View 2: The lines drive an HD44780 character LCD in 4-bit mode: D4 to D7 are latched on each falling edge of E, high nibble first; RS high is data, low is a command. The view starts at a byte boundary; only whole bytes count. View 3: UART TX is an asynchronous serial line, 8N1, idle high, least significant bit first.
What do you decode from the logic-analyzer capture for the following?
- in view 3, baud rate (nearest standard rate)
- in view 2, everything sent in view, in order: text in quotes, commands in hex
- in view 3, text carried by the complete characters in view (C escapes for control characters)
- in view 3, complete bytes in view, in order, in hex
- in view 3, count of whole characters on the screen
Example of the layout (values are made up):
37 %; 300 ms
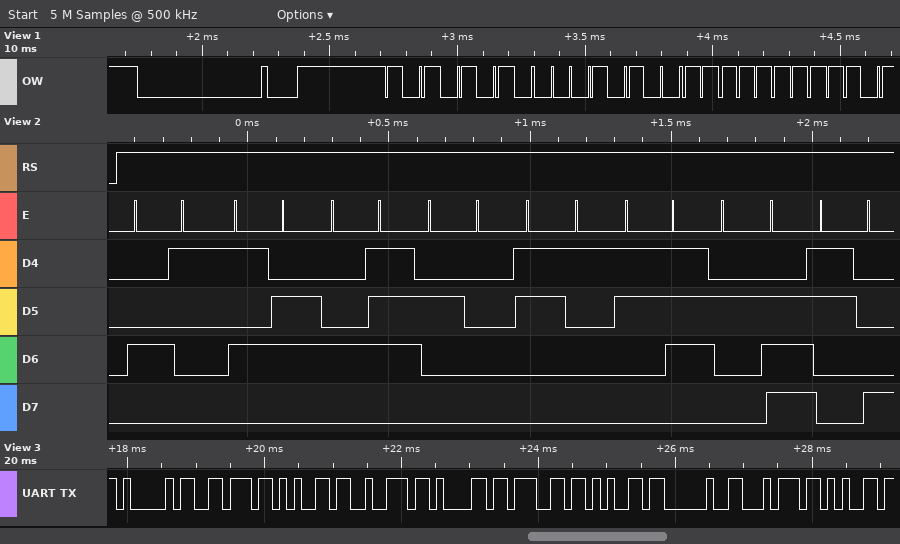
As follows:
9600 baud; "AVG 17.8"; "Average te"; 41 76 65 72 61 67 65 20 74 65; 10
